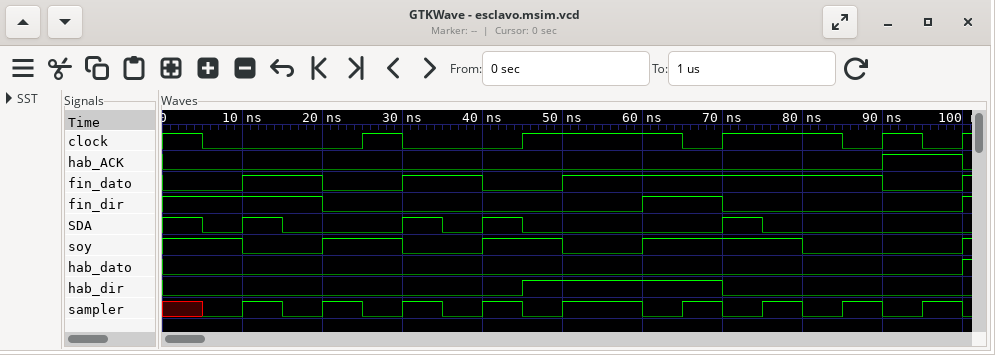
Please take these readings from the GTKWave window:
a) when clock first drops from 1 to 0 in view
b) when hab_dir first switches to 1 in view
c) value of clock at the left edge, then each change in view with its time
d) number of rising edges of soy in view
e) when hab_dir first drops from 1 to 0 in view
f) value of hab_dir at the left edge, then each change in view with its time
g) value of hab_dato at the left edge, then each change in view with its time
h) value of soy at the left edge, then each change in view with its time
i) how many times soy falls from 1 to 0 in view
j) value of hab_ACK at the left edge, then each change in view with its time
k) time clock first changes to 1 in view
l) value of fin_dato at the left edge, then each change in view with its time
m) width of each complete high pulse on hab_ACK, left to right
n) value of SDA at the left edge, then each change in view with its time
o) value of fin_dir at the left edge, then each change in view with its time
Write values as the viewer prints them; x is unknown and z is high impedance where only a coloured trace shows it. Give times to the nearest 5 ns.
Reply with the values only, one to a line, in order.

5 ns
45 ns
1, 0 at 5 ns, 1 at 25 ns, 0 at 30 ns, 1 at 45 ns, 0 at 65 ns, 1 at 70 ns, 0 at 85 ns, 1 at 90 ns, 0 at 95 ns, 1 at 100 ns
4
70 ns
0, 1 at 45 ns, 0 at 70 ns
0, 1 at 100 ns
1, 0 at 10 ns, 1 at 20 ns, 0 at 30 ns, 1 at 40 ns, 0 at 50 ns, 1 at 60 ns, 0 at 80 ns, 1 at 100 ns
4
0, 1 at 90 ns, 0 at 100 ns
25 ns
0, 1 at 10 ns, 0 at 20 ns, 1 at 30 ns, 0 at 40 ns, 1 at 50 ns, 0 at 90 ns, 1 at 100 ns
10 ns
1, 0 at 5 ns, 1 at 10 ns, 0 at 15 ns, 1 at 30 ns, 0 at 35 ns, 1 at 40 ns, 0 at 45 ns, 1 at 70 ns, 0 at 75 ns
1, 0 at 20 ns, 1 at 60 ns, 0 at 70 ns, 1 at 100 ns
